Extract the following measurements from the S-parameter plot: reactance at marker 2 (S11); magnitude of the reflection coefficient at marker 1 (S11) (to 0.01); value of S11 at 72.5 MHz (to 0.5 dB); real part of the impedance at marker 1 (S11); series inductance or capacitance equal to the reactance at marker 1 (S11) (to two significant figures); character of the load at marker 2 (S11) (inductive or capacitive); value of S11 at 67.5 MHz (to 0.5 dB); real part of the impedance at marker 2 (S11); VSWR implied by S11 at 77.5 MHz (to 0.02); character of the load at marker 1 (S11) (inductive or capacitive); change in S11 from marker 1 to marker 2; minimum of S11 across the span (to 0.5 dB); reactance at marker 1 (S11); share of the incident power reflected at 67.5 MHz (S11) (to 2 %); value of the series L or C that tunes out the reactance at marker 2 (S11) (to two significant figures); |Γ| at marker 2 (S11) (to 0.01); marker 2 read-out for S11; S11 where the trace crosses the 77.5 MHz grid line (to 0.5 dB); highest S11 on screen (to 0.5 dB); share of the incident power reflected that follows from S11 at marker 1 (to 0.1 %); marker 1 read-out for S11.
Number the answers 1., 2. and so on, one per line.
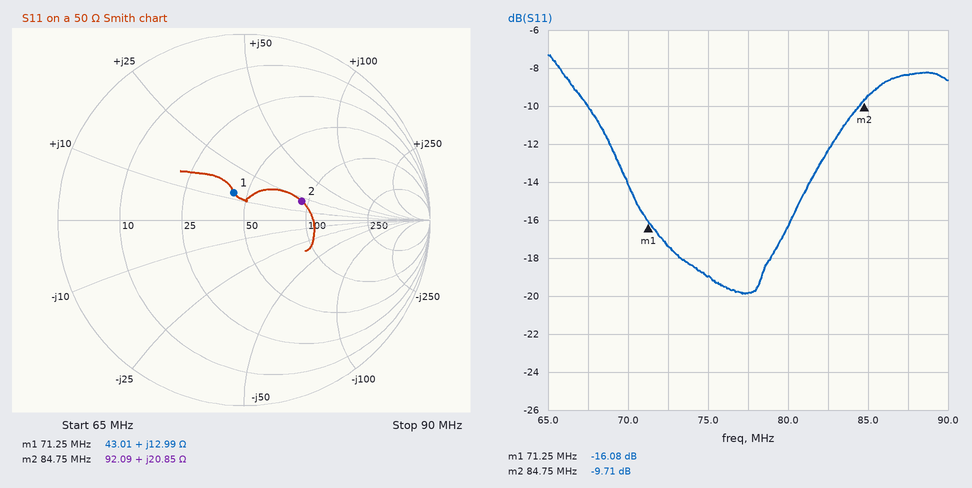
1. +20.85 Ω
2. 0.16
3. -17.5 dB
4. 43.01 Ω
5. 29 nH
6. inductive
7. -10.0 dB
8. 92.09 Ω
9. 1.22
10. inductive
11. 6.37 dB
12. -20.0 dB
13. +12.99 Ω
14. 10 %
15. 90 pF
16. 0.33
17. -9.71 dB
18. -20.0 dB
19. -7.5 dB
20. 2.5 %
21. -16.08 dB
